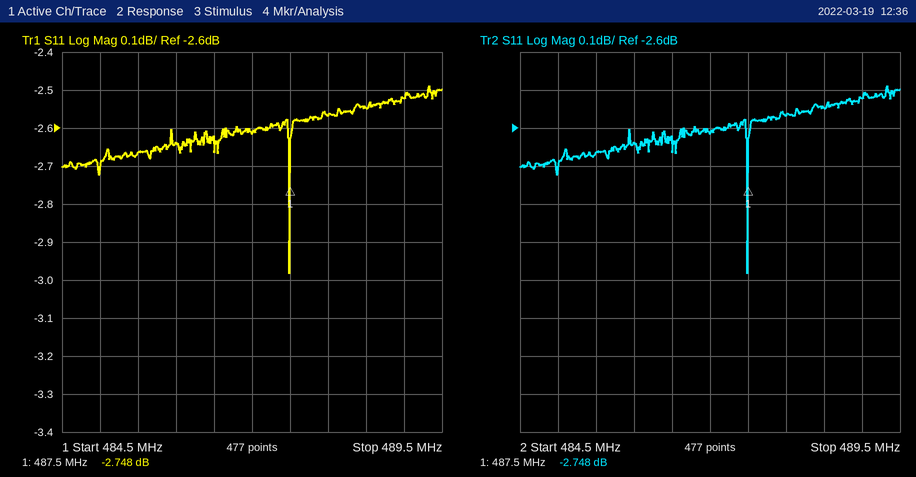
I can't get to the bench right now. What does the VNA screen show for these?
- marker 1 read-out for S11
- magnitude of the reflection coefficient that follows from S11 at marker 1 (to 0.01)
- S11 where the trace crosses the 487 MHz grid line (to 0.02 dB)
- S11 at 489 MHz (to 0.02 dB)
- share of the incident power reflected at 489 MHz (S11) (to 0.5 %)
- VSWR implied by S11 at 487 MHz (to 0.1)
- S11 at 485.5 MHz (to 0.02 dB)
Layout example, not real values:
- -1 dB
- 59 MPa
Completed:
- -2.748 dB
- 0.73
- -2.62 dB
- -2.52 dB
- 56.0 %
- 6.7
- -2.66 dB
